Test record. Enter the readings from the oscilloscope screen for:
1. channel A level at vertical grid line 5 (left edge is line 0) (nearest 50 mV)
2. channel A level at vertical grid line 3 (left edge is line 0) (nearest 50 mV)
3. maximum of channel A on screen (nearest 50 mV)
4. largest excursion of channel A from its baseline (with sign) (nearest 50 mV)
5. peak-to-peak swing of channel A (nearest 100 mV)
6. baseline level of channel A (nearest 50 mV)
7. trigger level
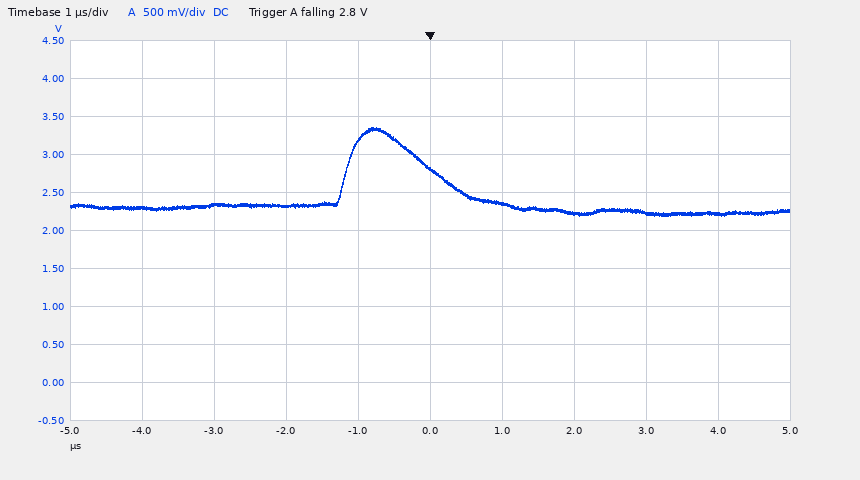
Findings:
2.80 V
2.30 V
3.35 V
+1.05 V
1.20 V
2.30 V
2.8 V
